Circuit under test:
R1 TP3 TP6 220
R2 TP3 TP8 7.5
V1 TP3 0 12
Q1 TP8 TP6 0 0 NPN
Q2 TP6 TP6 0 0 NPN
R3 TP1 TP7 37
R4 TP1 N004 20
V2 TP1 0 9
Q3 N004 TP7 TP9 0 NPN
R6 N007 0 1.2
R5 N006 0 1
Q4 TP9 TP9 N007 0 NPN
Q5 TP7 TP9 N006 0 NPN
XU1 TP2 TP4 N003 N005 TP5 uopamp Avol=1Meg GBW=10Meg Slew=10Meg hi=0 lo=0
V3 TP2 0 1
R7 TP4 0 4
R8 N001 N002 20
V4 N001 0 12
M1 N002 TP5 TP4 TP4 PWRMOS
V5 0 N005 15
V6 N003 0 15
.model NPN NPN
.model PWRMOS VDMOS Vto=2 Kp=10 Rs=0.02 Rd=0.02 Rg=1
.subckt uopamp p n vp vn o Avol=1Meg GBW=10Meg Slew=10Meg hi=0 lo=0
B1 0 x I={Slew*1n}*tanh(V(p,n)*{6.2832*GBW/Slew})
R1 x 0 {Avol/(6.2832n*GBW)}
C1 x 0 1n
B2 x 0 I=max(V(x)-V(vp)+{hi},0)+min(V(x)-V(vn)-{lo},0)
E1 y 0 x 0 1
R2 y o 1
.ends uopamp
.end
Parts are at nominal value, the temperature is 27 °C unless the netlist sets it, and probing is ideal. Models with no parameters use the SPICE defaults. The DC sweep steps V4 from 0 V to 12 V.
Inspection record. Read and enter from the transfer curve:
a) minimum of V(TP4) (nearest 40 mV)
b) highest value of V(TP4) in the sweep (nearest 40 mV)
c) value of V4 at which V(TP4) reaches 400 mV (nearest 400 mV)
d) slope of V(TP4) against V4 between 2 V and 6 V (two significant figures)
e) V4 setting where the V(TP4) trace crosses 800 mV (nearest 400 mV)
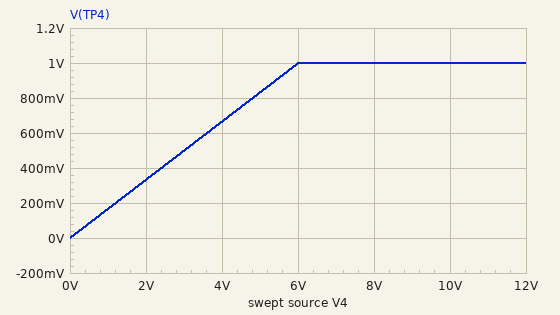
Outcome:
0 V
1.00 V
2.4 V
0.17 V/V
4.8 V
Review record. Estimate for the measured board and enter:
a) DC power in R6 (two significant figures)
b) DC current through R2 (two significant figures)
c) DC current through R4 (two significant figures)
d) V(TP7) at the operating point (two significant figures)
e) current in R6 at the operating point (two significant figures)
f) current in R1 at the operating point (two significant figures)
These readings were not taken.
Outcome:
31 mW
50 mA
160 mA
2.0 V
160 mA
51 mA
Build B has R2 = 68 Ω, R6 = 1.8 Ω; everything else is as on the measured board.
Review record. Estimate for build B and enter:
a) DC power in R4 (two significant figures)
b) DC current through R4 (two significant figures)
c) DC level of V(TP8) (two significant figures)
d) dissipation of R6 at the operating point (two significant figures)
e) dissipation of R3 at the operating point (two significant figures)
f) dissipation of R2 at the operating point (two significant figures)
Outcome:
260 mW
110 mA
8.6 V
23 mW
1.3 W
170 mW
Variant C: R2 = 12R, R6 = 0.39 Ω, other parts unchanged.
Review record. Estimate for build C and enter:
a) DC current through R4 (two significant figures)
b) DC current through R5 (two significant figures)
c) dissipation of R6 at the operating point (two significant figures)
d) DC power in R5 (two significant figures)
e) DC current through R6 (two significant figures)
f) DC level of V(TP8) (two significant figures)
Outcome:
390 mA
180 mA
63 mW
32 mW
400 mA
11 V
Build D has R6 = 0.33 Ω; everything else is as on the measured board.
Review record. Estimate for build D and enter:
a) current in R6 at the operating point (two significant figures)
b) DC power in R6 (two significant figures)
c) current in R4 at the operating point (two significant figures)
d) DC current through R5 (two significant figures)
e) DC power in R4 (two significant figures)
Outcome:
420 mA
58 mW
390 mA
160 mA
3.1 W
